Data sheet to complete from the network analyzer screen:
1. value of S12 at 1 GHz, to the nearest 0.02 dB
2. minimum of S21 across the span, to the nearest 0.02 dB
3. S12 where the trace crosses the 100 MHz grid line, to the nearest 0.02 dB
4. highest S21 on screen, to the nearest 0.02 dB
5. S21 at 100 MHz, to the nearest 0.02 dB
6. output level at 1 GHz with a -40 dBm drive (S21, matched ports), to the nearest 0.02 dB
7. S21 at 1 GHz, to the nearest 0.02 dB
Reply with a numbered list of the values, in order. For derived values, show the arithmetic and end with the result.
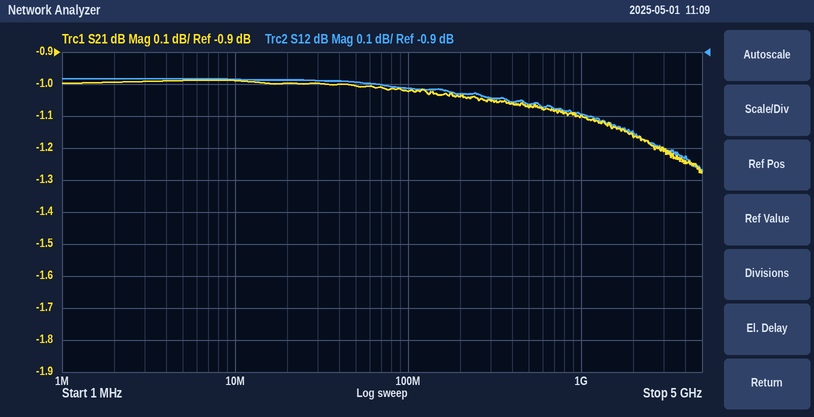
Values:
1. -1.10 dB
2. -1.28 dB
3. -1.02 dB
4. -0.98 dB
5. -1.02 dB
6. -40 dBm + (-1.10 dB) = -41.10 dBm
7. -1.10 dB
